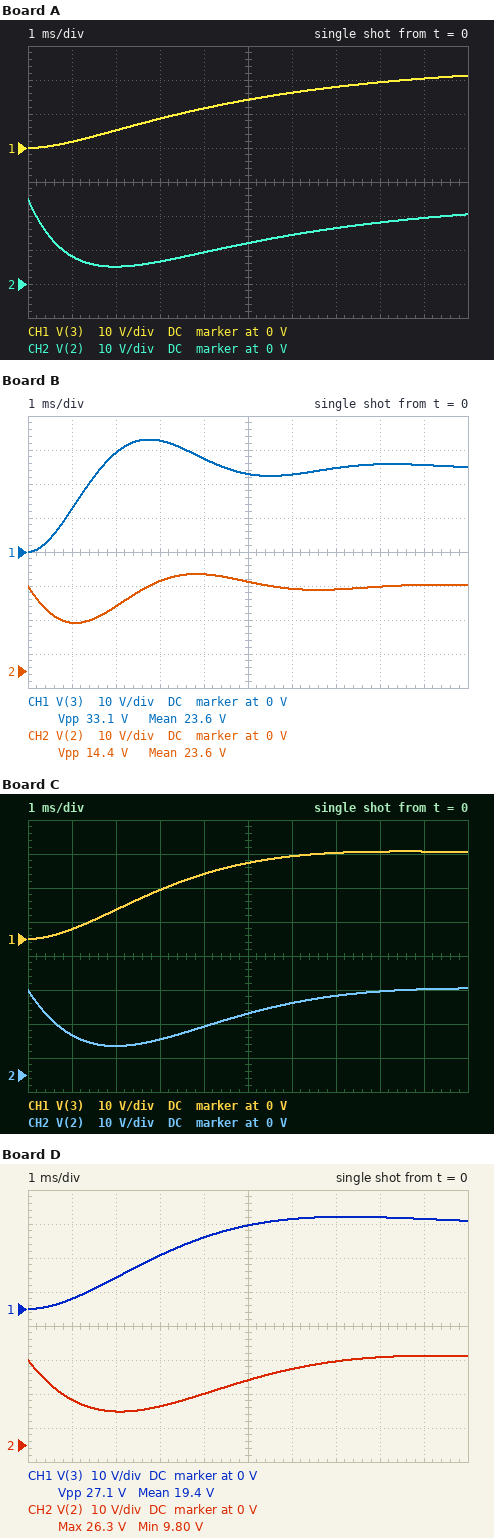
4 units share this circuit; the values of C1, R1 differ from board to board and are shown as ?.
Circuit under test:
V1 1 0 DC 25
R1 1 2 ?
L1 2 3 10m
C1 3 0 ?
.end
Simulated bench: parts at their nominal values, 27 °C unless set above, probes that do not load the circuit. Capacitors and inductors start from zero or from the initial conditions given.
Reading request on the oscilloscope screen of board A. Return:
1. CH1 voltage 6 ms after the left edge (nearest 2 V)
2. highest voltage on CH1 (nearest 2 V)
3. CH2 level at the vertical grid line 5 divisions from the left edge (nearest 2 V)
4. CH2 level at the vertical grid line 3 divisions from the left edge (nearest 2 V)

16 V
22 V
12 V
6 V
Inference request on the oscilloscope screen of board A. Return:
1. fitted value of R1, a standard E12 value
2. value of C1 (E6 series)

12 Ω
470 µF
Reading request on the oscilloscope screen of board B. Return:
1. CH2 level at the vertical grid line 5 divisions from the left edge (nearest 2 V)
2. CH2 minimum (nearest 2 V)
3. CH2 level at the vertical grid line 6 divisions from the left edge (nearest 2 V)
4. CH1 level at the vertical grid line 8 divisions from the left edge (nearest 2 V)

26 V
14 V
24 V
26 V
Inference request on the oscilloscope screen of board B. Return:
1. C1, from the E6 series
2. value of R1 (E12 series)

68 µF
8.2 Ω
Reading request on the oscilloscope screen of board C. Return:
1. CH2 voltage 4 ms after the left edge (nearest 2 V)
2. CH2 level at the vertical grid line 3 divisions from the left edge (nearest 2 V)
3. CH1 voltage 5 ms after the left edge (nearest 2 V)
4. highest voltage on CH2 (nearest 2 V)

14 V
10 V
22 V
26 V
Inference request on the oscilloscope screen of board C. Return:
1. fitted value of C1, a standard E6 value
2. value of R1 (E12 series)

330 µF
8.2 Ω
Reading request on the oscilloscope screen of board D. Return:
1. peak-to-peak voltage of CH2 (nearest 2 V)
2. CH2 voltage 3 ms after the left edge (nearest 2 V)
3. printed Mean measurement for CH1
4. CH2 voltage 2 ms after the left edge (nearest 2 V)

16 V
12 V
19.4 V
10 V
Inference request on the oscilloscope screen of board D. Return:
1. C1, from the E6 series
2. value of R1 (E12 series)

330 µF
6.8 Ω
